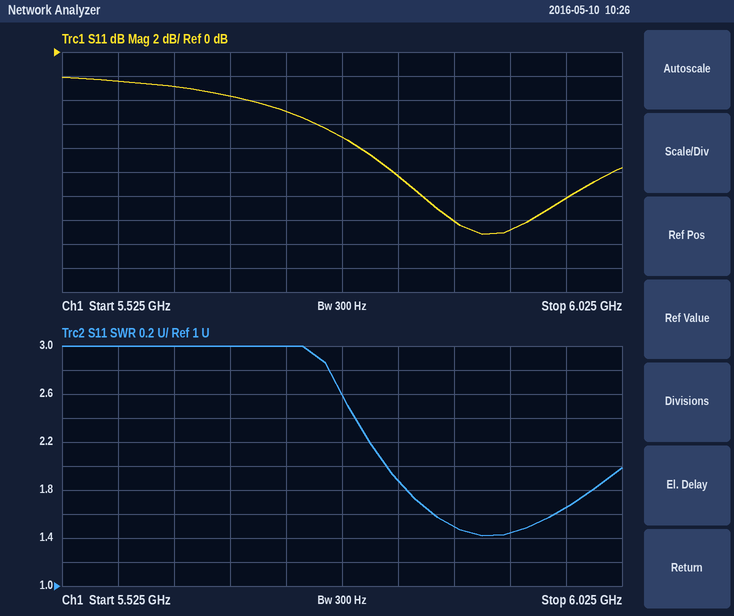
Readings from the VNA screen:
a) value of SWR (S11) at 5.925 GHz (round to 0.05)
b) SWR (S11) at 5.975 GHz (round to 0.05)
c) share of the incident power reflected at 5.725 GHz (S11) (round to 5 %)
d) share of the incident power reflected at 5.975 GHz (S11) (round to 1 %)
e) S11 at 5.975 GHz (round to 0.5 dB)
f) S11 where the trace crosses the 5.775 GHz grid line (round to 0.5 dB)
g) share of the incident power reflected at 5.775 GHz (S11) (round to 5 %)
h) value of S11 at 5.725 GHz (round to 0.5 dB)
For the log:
1.45
1.65
30 %
6 %
-12.0 dB
-7.0 dB
20 %
-5.0 dB
